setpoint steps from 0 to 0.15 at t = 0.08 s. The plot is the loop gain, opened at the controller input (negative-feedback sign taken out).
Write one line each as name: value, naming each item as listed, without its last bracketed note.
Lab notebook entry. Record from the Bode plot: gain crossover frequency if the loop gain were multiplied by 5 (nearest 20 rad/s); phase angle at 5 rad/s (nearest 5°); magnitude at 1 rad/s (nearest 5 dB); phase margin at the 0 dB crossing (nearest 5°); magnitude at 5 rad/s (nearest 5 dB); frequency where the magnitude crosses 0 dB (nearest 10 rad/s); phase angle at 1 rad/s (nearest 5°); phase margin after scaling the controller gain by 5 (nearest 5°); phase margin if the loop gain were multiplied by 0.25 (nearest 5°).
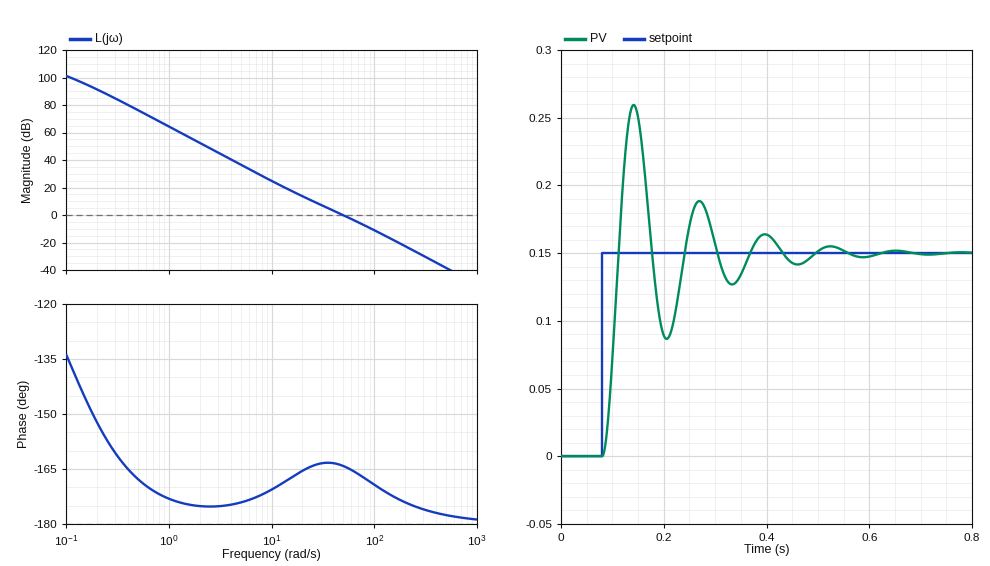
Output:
gain crossover frequency if the loop gain were multiplied by 5: 120 rad/s
phase angle at 5 rad/s: -175°
magnitude at 1 rad/s: 65 dB
phase margin at the 0 dB crossing: 15°
magnitude at 5 rad/s: 35 dB
frequency where the magnitude crosses 0 dB: 50 rad/s
phase angle at 1 rad/s: -175°
phase margin after scaling the controller gain by 5: 10°
phase margin if the loop gain were multiplied by 0.25: 15°
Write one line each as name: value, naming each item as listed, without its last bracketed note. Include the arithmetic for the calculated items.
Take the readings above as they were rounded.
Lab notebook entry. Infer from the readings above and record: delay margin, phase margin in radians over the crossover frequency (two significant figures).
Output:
delay margin, phase margin in radians over the crossover frequency: 15 × π / 180 / 50 = 0.0052 s
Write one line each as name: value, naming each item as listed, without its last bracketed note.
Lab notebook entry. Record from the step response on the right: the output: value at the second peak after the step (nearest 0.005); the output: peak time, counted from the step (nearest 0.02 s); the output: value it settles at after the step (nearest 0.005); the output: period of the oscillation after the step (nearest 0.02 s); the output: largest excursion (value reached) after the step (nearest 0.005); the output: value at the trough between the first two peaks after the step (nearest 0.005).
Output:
the output: value at the second peak after the step: 0.190
the output: peak time, counted from the step: 0.06 s
the output: value it settles at after the step: 0.150
the output: period of the oscillation after the step: 0.12 s
the output: largest excursion (value reached) after the step: 0.260
the output: value at the trough between the first two peaks after the step: 0.085
